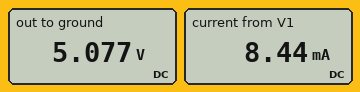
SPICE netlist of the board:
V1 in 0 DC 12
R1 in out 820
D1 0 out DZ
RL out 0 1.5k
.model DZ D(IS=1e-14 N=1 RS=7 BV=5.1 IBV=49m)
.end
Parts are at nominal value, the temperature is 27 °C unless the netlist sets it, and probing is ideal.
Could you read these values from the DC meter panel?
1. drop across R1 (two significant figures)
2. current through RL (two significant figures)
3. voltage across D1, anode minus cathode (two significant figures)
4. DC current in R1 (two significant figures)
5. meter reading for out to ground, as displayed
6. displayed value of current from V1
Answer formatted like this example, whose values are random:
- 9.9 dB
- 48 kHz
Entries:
- 6.9 V
- 3.4 mA
- -5.1 V
- 8.4 mA
- 5.077 V
- 8.44 mA
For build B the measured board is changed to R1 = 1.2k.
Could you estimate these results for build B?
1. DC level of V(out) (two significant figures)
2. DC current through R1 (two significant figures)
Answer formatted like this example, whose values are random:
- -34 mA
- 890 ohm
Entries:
- 5.0 V
- 5.8 mA
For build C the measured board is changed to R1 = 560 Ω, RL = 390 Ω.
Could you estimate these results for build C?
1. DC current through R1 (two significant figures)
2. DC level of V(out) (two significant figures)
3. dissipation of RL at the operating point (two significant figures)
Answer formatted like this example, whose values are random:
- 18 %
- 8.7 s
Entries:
- 13 mA
- 4.9 V
- 62 mW
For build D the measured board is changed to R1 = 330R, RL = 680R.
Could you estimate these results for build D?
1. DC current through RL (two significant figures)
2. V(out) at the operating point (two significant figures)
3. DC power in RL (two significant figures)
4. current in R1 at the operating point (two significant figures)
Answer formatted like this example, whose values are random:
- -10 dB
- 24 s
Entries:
- 7.6 mA
- 5.2 V
- 39 mW
- 21 mA
